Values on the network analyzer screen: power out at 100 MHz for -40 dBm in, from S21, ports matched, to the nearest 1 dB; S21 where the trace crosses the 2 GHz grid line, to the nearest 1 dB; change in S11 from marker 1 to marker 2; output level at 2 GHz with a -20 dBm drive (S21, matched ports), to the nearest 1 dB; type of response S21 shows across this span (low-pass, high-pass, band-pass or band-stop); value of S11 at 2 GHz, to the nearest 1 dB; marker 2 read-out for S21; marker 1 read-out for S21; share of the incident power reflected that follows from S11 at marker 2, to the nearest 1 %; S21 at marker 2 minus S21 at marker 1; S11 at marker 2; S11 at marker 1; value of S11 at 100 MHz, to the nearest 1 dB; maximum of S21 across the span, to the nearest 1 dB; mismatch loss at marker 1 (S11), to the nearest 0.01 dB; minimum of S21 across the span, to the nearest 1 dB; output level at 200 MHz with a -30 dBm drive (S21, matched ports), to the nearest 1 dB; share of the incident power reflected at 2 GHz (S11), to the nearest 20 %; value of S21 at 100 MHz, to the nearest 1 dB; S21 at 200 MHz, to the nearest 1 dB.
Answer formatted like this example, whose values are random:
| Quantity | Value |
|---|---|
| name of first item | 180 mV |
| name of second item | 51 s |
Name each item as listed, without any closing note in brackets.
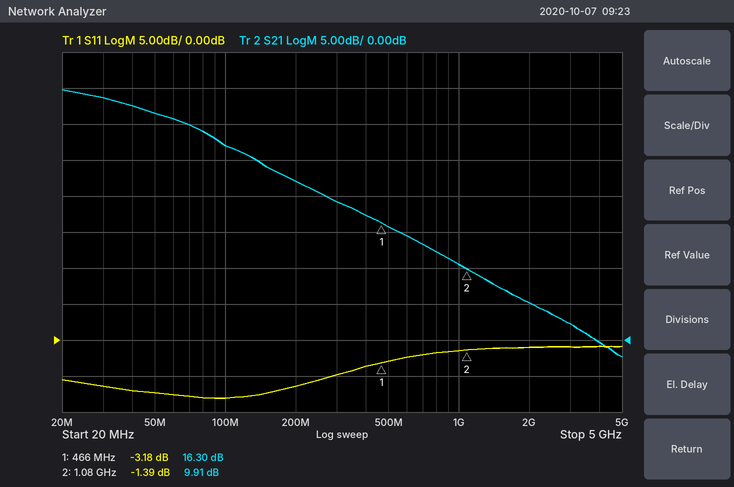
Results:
| Quantity | Value |
|---|---|
| power out at 100 MHz for -40 dBm in, from S21, ports matched, to the nearest 1 dB | -13 dBm |
| S21 where the trace crosses the 2 GHz grid line, to the nearest 1 dB | 5 dB |
| change in S11 from marker 1 to marker 2 | 1.79 dB |
| output level at 2 GHz with a -20 dBm drive (S21, matched ports), to the nearest 1 dB | -15 dBm |
| type of response S21 shows across this span | low-pass |
| value of S11 at 2 GHz, to the nearest 1 dB | -1 dB |
| marker 2 read-out for S21 | 9.91 dB |
| marker 1 read-out for S21 | 16.30 dB |
| share of the incident power reflected that follows from S11 at marker 2, to the nearest 1 % | 73 % |
| S21 at marker 2 minus S21 at marker 1 | -6.39 dB |
| S11 at marker 2 | -1.39 dB |
| S11 at marker 1 | -3.18 dB |
| value of S11 at 100 MHz, to the nearest 1 dB | -8 dB |
| maximum of S21 across the span, to the nearest 1 dB | 35 dB |
| mismatch loss at marker 1 (S11), to the nearest 0.01 dB | 2.85 dB |
| minimum of S21 across the span, to the nearest 1 dB | -2 dB |
| output level at 200 MHz with a -30 dBm drive (S21, matched ports), to the nearest 1 dB | -8 dBm |
| share of the incident power reflected at 2 GHz (S11), to the nearest 20 % | 80 % |
| value of S21 at 100 MHz, to the nearest 1 dB | 27 dB |
| S21 at 200 MHz, to the nearest 1 dB | 22 dB |
